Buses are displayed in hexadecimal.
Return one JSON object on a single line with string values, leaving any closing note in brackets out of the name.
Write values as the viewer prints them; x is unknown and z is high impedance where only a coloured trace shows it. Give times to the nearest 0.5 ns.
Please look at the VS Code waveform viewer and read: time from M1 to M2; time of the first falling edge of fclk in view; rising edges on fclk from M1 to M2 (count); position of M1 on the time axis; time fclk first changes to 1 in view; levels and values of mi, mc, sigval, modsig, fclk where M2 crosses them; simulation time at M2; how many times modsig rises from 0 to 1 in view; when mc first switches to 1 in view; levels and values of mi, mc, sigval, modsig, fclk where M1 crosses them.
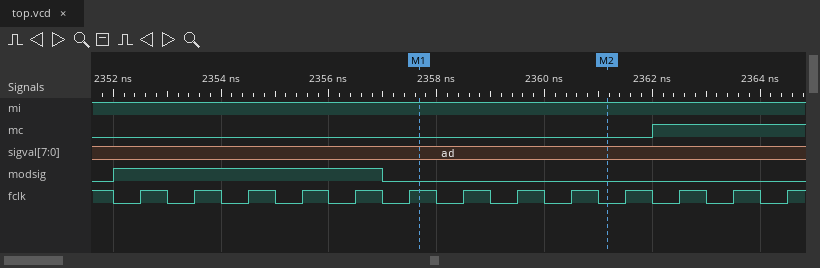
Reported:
{"time from M1 to M2": "3.5 ns", "time of the first falling edge of fclk in view": "2352 ns", "rising edges on fclk from M1 to M2": "3", "position of M1 on the time axis": "2357.5 ns", "time fclk first changes to 1 in view": "2352.5 ns", "levels and values of mi, mc, sigval, modsig, fclk where M2 crosses them": "mi=1, mc=0, sigval=ad, modsig=0, fclk=0", "simulation time at M2": "2361 ns", "how many times modsig rises from 0 to 1 in view": "1", "when mc first switches to 1 in view": "2362 ns", "levels and values of mi, mc, sigval, modsig, fclk where M1 crosses them": "mi=1, mc=0, sigval=ad, modsig=0, fclk=1"}
